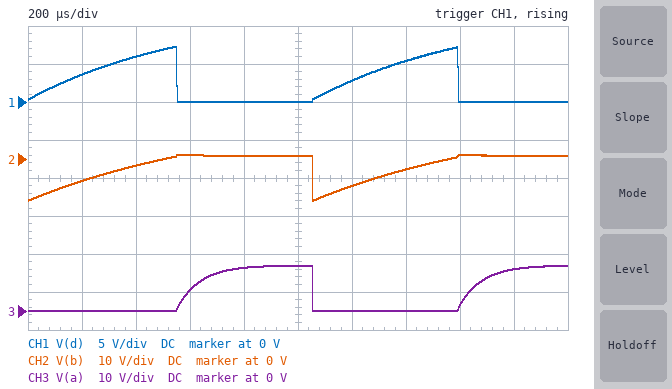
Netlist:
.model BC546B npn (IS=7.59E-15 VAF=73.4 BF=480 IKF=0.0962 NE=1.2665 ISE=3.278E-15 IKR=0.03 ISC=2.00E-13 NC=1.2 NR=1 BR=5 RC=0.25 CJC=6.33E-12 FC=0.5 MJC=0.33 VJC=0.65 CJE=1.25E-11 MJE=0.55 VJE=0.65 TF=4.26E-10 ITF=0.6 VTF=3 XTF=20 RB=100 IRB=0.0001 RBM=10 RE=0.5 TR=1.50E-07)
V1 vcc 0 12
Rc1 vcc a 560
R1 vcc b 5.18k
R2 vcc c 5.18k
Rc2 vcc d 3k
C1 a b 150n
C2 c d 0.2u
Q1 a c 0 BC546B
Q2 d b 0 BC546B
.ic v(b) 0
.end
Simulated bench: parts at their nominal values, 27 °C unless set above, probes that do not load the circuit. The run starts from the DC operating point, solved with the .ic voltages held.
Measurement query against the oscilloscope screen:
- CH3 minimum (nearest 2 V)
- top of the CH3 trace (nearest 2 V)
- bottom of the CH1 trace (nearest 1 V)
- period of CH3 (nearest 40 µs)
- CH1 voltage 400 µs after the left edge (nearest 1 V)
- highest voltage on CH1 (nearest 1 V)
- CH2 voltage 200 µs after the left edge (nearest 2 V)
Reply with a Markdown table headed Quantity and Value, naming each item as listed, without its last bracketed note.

| Quantity | Value |
|---|---|
| CH3 minimum | 0 V |
| top of the CH3 trace | 12 V |
| bottom of the CH1 trace | 0 V |
| period of CH3 | 1.04 ms |
| CH1 voltage 400 µs after the left edge | 6 V |
| highest voltage on CH1 | 7 V |
| CH2 voltage 200 µs after the left edge | -6 V |
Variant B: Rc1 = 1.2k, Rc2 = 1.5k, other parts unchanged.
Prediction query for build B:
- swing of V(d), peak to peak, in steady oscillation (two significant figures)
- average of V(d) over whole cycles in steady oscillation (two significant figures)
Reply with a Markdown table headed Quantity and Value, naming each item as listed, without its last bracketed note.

| Quantity | Value |
|---|---|
| swing of V(d), peak to peak, in steady oscillation | 10 V |
| average of V(d) over whole cycles in steady oscillation | 3.0 V |
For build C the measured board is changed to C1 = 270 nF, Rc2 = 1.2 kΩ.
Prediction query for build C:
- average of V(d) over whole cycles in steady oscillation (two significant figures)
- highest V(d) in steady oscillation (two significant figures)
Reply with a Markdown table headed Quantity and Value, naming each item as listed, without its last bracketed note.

| Quantity | Value |
|---|---|
| average of V(d) over whole cycles in steady oscillation | 5.3 V |
| highest V(d) in steady oscillation | 12 V |
